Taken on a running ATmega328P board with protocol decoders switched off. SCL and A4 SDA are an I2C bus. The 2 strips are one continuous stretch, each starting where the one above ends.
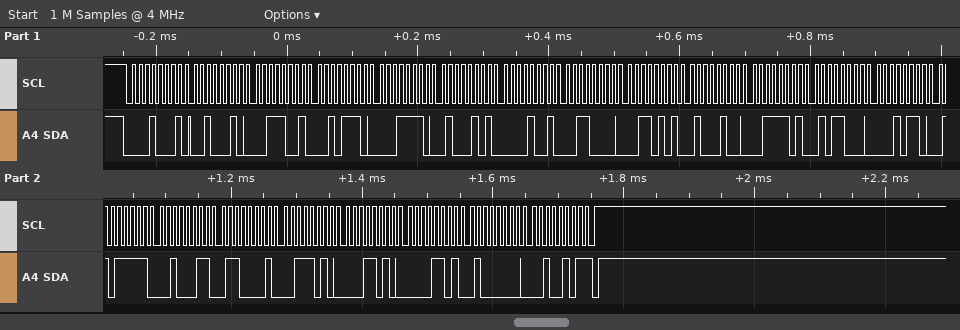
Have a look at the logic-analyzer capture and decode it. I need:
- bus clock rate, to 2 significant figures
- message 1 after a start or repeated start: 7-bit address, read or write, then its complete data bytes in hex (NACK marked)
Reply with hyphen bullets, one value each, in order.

- 100 kHz
- 0x08 read: 22 39 2E 1E 45 09 30 35 44 3D 58 16 5F 23 61 3A 1A 0D 40 25 NACK
